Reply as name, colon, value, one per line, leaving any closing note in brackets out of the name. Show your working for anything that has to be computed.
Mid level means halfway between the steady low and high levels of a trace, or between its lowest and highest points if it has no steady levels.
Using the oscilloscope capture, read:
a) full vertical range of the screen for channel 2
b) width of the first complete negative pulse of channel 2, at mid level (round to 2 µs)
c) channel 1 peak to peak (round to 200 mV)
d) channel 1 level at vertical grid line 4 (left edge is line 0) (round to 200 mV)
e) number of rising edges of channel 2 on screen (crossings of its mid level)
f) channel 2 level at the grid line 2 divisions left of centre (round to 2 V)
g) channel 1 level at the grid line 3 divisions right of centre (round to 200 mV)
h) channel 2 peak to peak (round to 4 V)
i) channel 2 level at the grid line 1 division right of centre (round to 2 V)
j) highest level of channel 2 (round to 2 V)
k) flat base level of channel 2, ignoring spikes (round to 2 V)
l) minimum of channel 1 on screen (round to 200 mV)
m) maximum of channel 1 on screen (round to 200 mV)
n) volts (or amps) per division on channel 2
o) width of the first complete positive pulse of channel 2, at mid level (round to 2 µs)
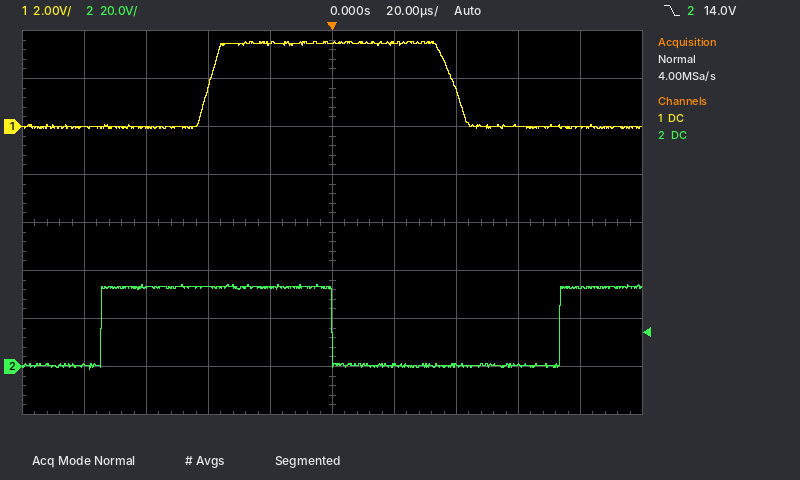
full vertical range of the screen for channel 2: 160 V
width of the first complete negative pulse of channel 2, at mid level: 74 µs
channel 1 peak to peak: 3.6 V − (0.0 V) = 3.6 V
channel 1 level at vertical grid line 4 (left edge is line 0): 3.4 V
number of rising edges of channel 2 on screen: 2
channel 2 level at the grid line 2 divisions left of centre: 34 V
channel 1 level at the grid line 3 divisions right of centre: 0.0 V
channel 2 peak to peak: 36 V
channel 2 level at the grid line 1 division right of centre: 0 V
highest level of channel 2: 34 V
flat base level of channel 2, ignoring spikes: 0 V
minimum of channel 1 on screen: 0.0 V
maximum of channel 1 on screen: 3.6 V
volts (or amps) per division on channel 2: 20 V
width of the first complete positive pulse of channel 2, at mid level: 74 µs
